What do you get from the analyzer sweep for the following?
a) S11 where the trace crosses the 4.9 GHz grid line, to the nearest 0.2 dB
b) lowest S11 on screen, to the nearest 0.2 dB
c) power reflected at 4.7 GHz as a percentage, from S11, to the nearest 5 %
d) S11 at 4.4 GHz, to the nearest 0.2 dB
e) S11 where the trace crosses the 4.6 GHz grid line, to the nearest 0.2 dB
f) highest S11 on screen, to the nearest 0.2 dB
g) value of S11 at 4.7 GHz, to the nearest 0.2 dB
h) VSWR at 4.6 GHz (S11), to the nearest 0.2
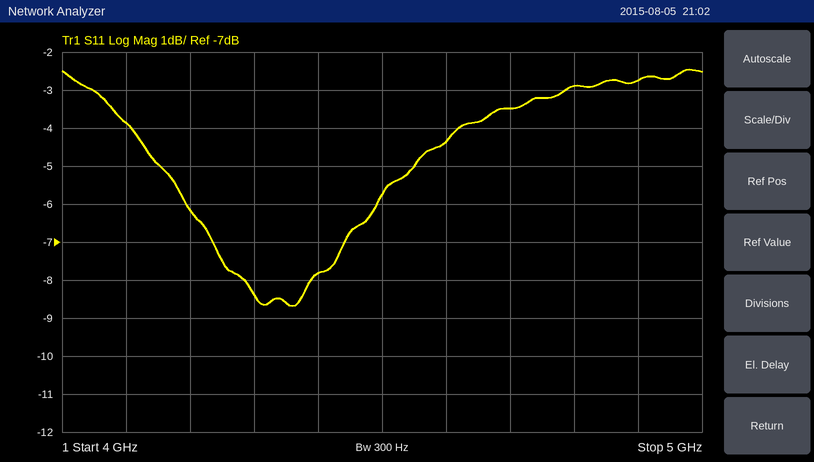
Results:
-2.8 dB
-8.6 dB
45 %
-7.8 dB
-4.4 dB
-2.4 dB
-3.4 dB
4.0
